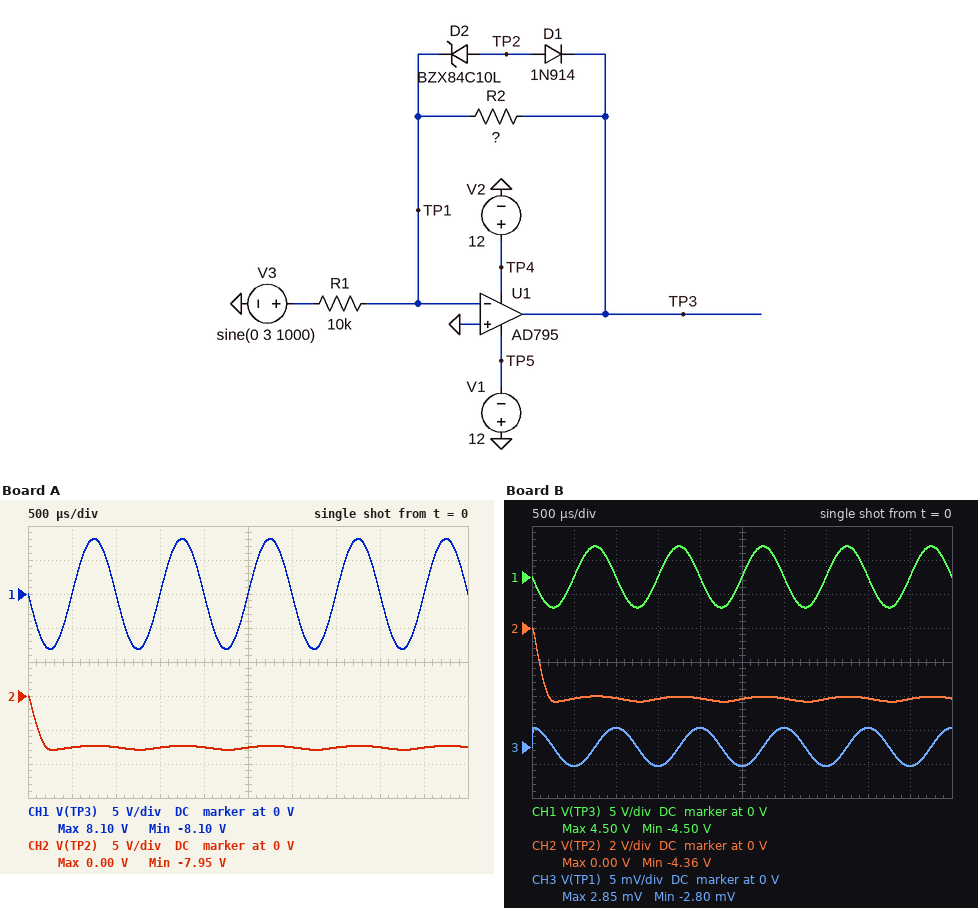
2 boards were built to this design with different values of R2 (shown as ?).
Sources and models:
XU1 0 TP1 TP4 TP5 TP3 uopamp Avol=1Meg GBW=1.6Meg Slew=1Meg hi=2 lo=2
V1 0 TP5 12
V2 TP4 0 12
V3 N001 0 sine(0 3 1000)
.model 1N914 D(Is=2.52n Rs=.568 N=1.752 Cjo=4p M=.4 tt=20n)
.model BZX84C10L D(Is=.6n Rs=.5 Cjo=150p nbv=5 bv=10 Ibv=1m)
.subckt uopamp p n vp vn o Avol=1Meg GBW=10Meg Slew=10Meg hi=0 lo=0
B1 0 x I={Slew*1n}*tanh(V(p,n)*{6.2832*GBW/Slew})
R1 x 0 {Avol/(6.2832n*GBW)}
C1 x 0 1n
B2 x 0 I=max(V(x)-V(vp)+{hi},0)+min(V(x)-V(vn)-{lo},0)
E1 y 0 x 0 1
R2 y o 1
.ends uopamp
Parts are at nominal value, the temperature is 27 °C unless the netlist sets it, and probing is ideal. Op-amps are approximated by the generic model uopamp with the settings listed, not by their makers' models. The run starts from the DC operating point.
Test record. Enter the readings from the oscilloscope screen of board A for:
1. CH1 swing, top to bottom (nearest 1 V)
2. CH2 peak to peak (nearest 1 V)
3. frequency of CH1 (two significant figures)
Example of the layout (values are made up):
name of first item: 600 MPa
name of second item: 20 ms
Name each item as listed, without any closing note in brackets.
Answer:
CH1 swing, top to bottom: 16 V
CH2 peak to peak: 8 V
frequency of CH1: 1.0 kHz
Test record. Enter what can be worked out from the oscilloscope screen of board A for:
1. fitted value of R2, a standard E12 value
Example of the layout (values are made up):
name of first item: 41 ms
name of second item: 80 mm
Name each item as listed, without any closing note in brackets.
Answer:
fitted value of R2, a standard E12 value: 27 kΩ
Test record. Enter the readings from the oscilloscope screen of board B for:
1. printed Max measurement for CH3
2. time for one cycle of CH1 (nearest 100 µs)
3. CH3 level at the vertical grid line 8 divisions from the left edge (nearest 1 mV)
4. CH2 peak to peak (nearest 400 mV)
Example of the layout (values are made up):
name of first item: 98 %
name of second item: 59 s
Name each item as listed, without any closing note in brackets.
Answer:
printed Max measurement for CH3: 2.85 mV
time for one cycle of CH1: 1.0 ms
CH3 level at the vertical grid line 8 divisions from the left edge: 3 mV
CH2 peak to peak: 4.4 V
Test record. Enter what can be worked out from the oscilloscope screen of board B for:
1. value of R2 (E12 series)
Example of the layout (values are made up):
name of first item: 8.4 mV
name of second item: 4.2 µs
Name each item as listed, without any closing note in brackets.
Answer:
value of R2: 15 kΩ
